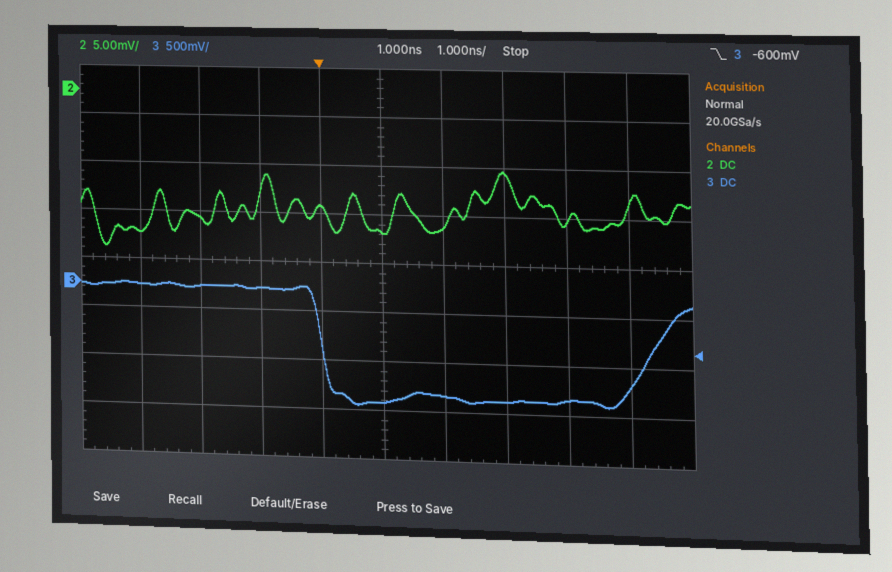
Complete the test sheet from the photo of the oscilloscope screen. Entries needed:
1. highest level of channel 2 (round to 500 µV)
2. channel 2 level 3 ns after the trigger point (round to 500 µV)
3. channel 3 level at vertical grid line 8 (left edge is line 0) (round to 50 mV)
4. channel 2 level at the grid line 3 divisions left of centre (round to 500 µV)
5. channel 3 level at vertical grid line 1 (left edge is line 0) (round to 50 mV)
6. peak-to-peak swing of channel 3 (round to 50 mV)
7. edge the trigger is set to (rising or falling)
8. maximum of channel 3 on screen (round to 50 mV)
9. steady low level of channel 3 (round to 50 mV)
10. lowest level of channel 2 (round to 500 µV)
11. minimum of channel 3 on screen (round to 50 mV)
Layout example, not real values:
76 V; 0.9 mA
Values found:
-8.0 mV; -8.0 mV; -1.10 V; -13.0 mV; 0 mV; 1.20 V; falling; 0 mV; -1.10 V; -16.0 mV; -1.20 V
